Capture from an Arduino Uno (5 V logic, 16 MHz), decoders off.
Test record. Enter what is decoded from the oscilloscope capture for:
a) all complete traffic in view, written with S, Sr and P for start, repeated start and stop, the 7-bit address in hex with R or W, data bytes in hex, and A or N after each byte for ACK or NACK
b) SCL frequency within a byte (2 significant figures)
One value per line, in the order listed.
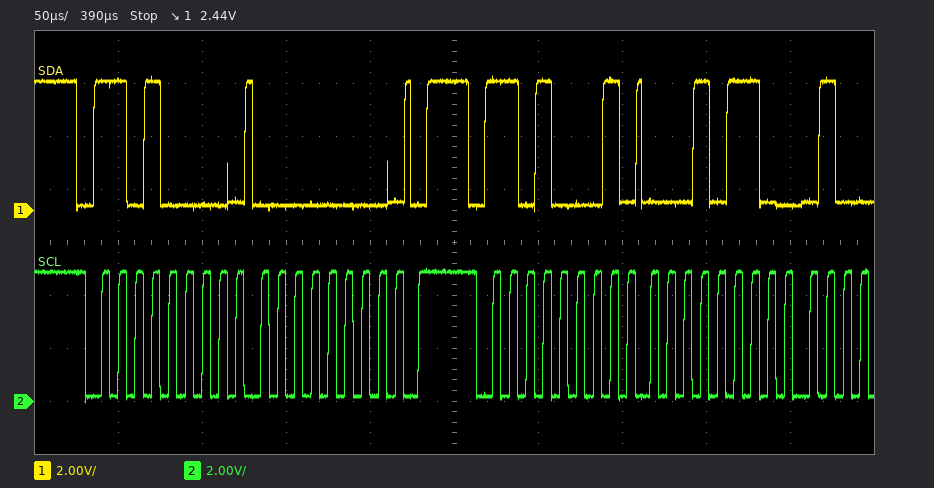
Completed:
S 68W A 00 A P S 68R A 16 A
100 kHz
